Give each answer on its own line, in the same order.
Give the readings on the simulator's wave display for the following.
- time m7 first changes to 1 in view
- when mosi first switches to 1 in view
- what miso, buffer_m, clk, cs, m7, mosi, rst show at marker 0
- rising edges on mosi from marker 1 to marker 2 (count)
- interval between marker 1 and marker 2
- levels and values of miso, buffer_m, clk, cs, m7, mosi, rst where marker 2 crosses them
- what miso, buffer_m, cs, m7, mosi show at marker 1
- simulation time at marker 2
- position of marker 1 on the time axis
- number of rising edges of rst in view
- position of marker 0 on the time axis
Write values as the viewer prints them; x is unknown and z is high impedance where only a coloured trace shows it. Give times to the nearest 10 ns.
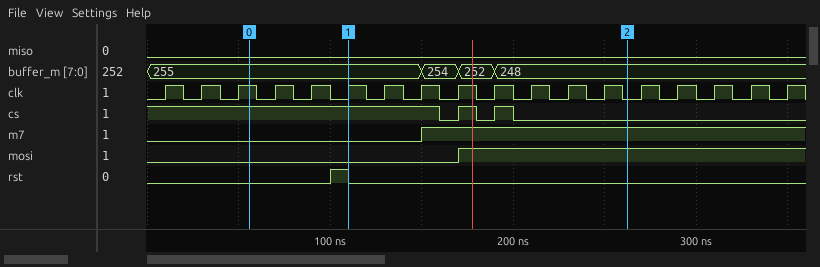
150 ns
170 ns
miso=0, buffer_m=255, clk=1, cs=1, m7=0, mosi=0, rst=0
1
150 ns
miso=0, buffer_m=248, clk=0, cs=0, m7=1, mosi=1, rst=0
miso=0, buffer_m=255, cs=1, m7=0, mosi=0
260 ns
110 ns
1
60 ns
